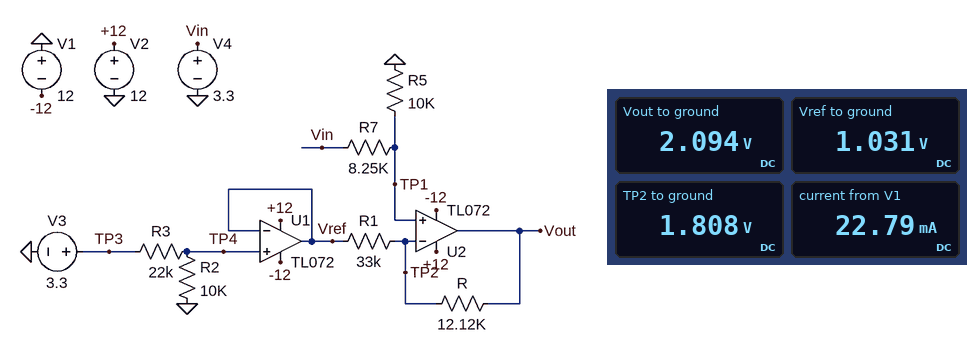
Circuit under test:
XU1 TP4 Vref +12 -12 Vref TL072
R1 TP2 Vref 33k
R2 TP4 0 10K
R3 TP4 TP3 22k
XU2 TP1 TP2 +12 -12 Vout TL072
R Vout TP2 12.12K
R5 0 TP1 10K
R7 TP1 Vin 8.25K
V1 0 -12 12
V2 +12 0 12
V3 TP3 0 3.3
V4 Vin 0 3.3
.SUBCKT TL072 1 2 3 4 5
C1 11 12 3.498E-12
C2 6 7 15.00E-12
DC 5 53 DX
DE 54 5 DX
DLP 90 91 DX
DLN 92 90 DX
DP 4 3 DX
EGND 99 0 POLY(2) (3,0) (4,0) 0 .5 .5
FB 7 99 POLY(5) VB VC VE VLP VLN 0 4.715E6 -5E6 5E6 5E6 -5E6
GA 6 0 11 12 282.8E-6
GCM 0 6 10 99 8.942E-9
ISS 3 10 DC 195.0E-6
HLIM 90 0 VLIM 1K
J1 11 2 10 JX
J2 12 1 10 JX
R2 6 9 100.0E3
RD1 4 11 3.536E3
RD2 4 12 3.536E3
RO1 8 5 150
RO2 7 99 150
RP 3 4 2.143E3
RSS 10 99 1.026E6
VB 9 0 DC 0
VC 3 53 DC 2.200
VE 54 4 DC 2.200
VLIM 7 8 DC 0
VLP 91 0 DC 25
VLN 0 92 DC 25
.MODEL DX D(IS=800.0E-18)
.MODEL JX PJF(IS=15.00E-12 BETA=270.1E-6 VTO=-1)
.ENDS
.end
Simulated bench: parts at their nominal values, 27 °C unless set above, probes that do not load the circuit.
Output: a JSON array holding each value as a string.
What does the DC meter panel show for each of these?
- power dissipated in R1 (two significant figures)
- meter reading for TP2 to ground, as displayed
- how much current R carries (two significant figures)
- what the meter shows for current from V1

["18 µW", "1.808 V", "24 µA", "22.79 mA"]
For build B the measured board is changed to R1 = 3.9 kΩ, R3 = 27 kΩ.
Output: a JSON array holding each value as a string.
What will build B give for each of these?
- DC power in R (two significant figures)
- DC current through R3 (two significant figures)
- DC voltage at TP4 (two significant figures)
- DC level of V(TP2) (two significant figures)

["670 µW", "89 µA", "890 mV", "1.8 V"]
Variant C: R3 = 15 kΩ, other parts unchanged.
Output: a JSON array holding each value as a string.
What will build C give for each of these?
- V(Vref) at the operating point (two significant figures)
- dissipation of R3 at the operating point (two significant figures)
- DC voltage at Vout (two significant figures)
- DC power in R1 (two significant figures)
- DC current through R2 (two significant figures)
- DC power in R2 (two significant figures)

["1.3 V", "260 µW", "2.0 V", "7.2 µW", "130 µA", "170 µW"]
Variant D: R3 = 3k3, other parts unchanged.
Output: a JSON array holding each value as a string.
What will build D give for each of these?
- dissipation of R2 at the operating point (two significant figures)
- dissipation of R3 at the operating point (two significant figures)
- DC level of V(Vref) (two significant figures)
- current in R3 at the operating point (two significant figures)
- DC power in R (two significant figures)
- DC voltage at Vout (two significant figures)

["620 µW", "200 µW", "2.5 V", "250 µA", "5.0 µW", "1.6 V"]
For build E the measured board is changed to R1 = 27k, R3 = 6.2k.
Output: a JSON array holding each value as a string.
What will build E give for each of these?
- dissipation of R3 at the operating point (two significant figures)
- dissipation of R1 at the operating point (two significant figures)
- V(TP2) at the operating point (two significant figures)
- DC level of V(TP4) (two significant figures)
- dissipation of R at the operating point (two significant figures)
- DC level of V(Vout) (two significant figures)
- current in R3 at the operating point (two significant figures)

["260 µW", "1.9 µW", "1.8 V", "2.0 V", "870 nW", "1.7 V", "200 µA"]
